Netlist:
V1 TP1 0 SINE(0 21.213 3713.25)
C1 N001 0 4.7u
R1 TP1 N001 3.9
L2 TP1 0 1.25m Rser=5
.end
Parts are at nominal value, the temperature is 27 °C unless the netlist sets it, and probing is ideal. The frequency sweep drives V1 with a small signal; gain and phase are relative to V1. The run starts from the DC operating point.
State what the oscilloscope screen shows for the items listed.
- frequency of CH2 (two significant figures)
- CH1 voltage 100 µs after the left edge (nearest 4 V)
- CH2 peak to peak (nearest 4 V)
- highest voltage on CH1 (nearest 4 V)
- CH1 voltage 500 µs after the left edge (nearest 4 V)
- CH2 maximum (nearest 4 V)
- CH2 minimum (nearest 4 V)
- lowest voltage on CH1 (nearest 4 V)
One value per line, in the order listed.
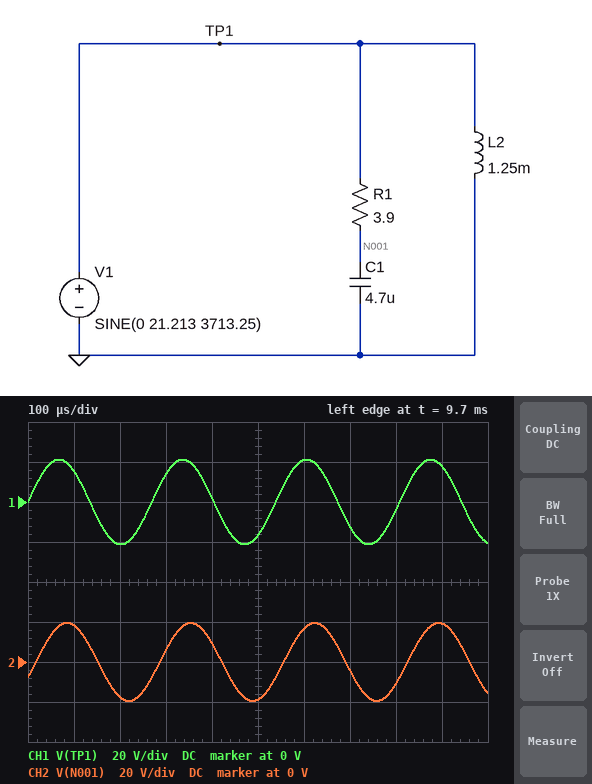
3.7 kHz
16 V
40 V
20 V
-16 V
20 V
-20 V
-20 V
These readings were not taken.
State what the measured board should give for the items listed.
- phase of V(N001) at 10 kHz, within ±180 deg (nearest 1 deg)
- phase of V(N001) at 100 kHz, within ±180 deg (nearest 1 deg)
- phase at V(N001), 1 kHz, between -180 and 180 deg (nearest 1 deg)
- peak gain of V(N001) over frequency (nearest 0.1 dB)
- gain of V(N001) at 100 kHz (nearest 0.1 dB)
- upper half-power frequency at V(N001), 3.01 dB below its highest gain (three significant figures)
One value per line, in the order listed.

-49 deg
-85 deg
-7 deg
0 dB
-21.3 dB
8.68 kHz
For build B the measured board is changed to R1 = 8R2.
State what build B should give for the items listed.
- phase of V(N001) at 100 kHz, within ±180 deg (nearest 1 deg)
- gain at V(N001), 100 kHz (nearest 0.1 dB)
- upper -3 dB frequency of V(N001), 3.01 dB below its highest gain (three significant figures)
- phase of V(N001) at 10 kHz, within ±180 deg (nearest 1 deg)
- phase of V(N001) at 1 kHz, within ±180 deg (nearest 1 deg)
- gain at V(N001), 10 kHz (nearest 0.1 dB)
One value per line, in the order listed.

-88 deg
-27.7 dB
4.13 kHz
-68 deg
-14 deg
-8.4 dB
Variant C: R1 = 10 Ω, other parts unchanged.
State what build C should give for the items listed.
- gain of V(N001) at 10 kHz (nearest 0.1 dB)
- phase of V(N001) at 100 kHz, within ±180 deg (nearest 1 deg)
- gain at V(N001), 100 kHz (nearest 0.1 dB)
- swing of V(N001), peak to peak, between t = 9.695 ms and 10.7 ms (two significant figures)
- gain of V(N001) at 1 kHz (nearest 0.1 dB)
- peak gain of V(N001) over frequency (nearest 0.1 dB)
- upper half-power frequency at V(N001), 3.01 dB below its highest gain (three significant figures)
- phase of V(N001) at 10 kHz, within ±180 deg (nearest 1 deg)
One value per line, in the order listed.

-9.9 dB
-88 deg
-29.4 dB
29 V
-0.4 dB
0 dB
3.39 kHz
-71 deg
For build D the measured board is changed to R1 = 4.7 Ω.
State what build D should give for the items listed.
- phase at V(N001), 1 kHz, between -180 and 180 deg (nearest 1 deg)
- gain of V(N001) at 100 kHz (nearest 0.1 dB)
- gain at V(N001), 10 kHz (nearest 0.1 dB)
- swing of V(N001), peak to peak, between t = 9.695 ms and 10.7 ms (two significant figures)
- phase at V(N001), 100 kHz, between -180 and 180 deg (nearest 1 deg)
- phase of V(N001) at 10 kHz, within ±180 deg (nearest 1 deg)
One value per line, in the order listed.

-8 deg
-22.9 dB
-4.7 dB
38 V
-86 deg
-54 deg
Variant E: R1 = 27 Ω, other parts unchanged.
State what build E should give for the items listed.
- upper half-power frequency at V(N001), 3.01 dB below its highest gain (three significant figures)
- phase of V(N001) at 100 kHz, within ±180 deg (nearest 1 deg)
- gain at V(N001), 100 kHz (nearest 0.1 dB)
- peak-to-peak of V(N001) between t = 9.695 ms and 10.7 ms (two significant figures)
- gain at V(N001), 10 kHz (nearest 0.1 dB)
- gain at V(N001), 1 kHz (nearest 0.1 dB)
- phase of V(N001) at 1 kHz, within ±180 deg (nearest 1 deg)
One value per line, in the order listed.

1.25 kHz
-89 deg
-38.0 dB
14 V
-18.1 dB
-2.1 dB
-39 deg
